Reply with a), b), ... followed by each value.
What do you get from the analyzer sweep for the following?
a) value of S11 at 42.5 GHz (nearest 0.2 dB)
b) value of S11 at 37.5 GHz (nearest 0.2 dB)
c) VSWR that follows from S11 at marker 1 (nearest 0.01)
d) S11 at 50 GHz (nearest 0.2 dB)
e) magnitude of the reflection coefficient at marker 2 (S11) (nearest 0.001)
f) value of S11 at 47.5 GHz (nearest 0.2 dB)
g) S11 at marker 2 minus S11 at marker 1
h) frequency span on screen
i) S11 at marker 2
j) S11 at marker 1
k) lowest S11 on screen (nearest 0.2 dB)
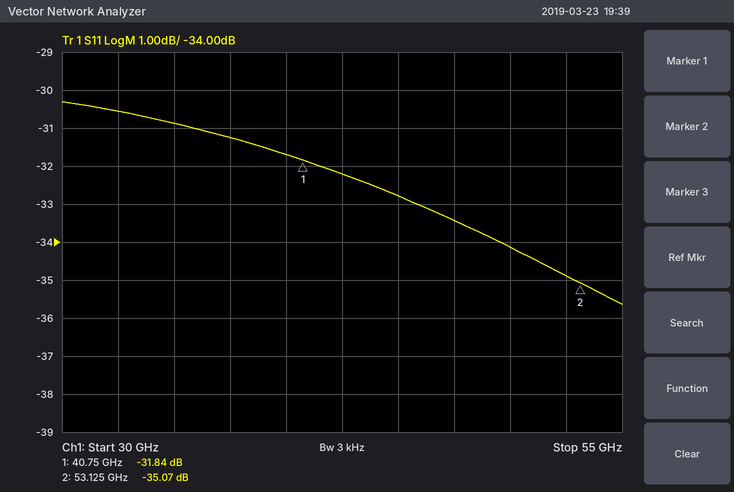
a) -32.2 dB
b) -31.2 dB
c) 1.05
d) -34.2 dB
e) 0.018
f) -33.4 dB
g) -3.23 dB
h) 25 GHz
i) -35.07 dB
j) -31.84 dB
k) -35.6 dB
